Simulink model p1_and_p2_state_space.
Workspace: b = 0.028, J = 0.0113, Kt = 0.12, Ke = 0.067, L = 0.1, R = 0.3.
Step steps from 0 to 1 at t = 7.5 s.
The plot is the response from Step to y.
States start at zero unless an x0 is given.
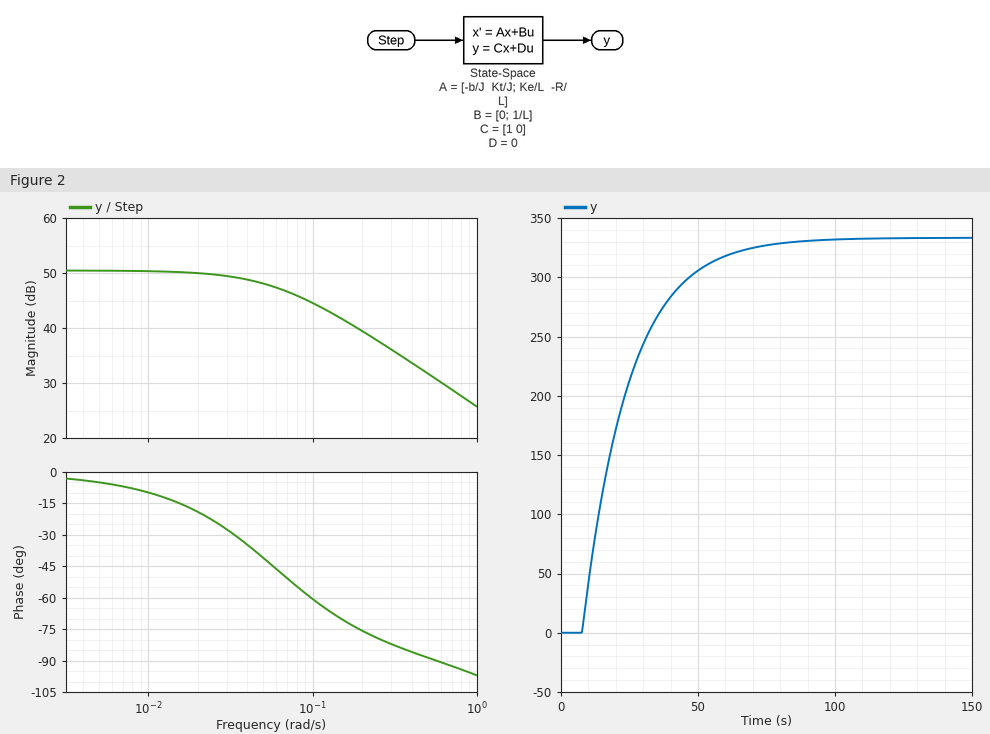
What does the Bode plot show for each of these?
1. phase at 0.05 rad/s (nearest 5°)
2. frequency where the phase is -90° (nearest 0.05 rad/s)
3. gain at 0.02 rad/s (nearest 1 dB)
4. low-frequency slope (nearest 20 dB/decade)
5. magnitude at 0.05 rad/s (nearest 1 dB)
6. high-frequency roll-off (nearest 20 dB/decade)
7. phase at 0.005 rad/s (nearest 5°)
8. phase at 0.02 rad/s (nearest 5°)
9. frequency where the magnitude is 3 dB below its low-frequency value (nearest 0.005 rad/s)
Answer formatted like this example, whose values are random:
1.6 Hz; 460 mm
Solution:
-40°; 0.55 rad/s; 50 dB; 0 dB/decade; 48 dB; -20 dB/decade; -5°; -20°; 0.060 rad/s
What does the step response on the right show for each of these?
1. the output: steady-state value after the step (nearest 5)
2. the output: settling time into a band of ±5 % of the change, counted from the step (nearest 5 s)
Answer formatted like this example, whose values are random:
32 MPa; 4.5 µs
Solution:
335; 50 s
